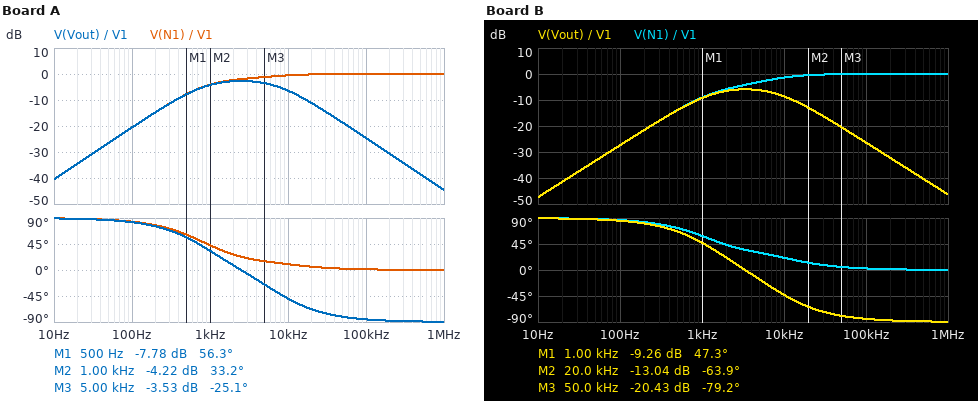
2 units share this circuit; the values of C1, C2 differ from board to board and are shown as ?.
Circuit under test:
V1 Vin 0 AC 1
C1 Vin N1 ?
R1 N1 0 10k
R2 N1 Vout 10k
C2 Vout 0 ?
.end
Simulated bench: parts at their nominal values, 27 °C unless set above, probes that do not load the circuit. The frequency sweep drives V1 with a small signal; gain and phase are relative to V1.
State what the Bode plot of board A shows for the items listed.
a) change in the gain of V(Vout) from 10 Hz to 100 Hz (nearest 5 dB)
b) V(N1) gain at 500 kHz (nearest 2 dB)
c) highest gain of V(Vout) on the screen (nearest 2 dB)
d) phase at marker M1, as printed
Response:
20 dB
0 dB
-2 dB
56.3 deg
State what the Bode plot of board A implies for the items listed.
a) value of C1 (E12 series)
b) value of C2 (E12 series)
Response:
15 nF
2.7 nF
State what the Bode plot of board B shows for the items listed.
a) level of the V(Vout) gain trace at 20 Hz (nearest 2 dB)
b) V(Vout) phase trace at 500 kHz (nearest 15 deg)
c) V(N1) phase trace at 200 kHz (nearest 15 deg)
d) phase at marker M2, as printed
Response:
-42 dB
-90 deg
0 deg
-63.9 deg
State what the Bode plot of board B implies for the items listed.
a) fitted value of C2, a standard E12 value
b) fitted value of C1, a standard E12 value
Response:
3.3 nF
6.8 nF
